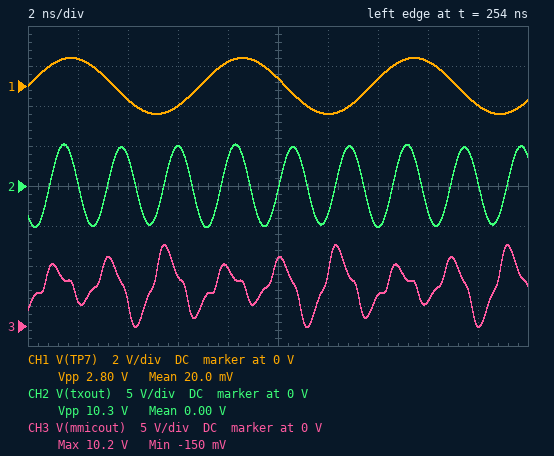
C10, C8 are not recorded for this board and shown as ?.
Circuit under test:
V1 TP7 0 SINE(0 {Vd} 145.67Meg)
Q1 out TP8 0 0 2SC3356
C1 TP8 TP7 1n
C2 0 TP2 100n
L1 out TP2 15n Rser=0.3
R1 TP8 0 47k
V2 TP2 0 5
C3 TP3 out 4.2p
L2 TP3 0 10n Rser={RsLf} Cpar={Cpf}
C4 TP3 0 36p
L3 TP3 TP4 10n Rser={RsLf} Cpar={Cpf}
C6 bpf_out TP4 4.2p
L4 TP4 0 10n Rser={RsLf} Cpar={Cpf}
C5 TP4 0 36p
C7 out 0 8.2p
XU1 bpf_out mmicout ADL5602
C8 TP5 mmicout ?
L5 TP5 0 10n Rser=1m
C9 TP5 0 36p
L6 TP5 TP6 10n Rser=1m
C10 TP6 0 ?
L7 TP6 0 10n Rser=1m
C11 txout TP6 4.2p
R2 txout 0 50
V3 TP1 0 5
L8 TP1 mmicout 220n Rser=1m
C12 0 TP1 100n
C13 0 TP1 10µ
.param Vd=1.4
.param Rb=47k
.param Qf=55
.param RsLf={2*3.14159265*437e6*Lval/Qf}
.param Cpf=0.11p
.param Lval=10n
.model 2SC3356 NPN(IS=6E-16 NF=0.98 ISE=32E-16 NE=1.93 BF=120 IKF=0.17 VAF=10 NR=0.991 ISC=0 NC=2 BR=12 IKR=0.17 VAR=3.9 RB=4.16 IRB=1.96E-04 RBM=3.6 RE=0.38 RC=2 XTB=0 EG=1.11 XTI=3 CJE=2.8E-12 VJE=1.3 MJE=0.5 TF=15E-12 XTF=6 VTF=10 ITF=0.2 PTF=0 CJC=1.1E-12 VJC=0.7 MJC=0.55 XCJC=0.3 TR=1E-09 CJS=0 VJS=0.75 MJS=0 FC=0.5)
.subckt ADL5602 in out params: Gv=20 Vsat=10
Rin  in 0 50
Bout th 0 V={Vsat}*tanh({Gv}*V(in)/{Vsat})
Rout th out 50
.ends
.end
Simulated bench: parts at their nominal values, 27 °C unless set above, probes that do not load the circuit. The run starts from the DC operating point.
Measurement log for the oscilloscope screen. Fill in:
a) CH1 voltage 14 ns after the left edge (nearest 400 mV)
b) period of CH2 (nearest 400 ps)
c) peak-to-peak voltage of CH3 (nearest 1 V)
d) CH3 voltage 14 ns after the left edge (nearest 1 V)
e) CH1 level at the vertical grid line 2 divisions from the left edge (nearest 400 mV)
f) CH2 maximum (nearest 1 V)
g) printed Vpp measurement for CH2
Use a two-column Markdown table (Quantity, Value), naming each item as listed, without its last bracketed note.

| Quantity | Value |
|---|---|
| CH1 voltage 14 ns after the left edge | 400 mV |
| period of CH2 | 2.4 ns |
| peak-to-peak voltage of CH3 | 10 V |
| CH3 voltage 14 ns after the left edge | 4 V |
| CH1 level at the vertical grid line 2 divisions from the left edge | -800 mV |
| CH2 maximum | 5 V |
| printed Vpp measurement for CH2 | 10.3 V |
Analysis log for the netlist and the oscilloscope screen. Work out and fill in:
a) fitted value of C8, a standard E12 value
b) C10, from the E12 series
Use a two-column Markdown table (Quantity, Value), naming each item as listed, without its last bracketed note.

| Quantity | Value |
|---|---|
| fitted value of C8, a standard E12 value | 12 pF |
| C10, from the E12 series | 33 pF |
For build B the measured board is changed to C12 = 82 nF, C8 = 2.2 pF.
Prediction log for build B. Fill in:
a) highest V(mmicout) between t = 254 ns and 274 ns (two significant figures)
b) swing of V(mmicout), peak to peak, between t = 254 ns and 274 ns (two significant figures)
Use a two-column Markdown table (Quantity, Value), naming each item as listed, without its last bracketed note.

| Quantity | Value |
|---|---|
| highest V(mmicout) between t = 254 ns and 274 ns | 15 V |
| swing of V(mmicout), peak to peak, between t = 254 ns and 274 ns | 19 V |
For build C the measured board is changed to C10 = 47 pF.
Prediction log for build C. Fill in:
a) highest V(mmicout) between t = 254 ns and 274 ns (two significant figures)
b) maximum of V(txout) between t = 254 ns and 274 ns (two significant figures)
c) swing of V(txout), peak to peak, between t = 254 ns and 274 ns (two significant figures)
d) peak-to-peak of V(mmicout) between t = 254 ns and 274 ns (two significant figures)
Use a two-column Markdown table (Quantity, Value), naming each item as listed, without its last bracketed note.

| Quantity | Value |
|---|---|
| highest V(mmicout) between t = 254 ns and 274 ns | 16 V |
| maximum of V(txout) between t = 254 ns and 274 ns | 2.8 V |
| swing of V(txout), peak to peak, between t = 254 ns and 274 ns | 5.5 V |
| peak-to-peak of V(mmicout) between t = 254 ns and 274 ns | 23 V |
